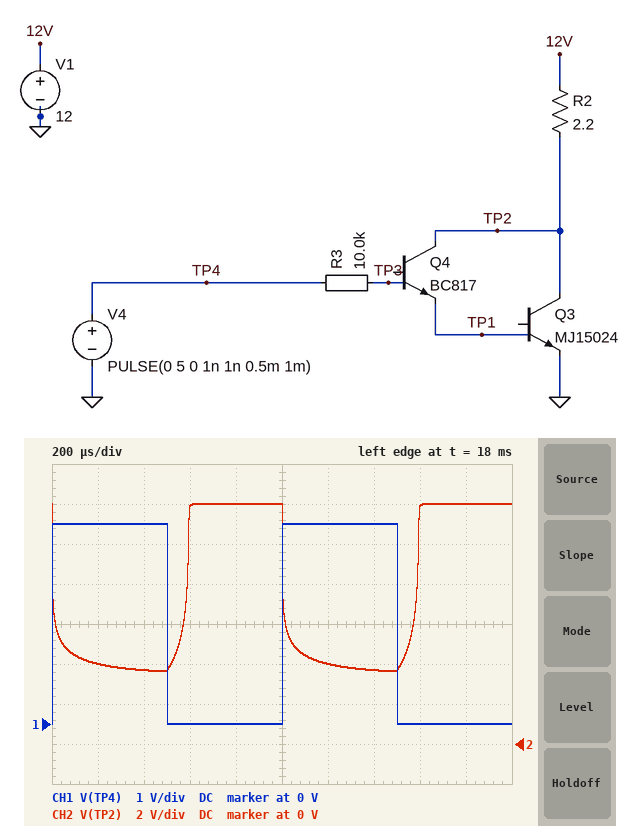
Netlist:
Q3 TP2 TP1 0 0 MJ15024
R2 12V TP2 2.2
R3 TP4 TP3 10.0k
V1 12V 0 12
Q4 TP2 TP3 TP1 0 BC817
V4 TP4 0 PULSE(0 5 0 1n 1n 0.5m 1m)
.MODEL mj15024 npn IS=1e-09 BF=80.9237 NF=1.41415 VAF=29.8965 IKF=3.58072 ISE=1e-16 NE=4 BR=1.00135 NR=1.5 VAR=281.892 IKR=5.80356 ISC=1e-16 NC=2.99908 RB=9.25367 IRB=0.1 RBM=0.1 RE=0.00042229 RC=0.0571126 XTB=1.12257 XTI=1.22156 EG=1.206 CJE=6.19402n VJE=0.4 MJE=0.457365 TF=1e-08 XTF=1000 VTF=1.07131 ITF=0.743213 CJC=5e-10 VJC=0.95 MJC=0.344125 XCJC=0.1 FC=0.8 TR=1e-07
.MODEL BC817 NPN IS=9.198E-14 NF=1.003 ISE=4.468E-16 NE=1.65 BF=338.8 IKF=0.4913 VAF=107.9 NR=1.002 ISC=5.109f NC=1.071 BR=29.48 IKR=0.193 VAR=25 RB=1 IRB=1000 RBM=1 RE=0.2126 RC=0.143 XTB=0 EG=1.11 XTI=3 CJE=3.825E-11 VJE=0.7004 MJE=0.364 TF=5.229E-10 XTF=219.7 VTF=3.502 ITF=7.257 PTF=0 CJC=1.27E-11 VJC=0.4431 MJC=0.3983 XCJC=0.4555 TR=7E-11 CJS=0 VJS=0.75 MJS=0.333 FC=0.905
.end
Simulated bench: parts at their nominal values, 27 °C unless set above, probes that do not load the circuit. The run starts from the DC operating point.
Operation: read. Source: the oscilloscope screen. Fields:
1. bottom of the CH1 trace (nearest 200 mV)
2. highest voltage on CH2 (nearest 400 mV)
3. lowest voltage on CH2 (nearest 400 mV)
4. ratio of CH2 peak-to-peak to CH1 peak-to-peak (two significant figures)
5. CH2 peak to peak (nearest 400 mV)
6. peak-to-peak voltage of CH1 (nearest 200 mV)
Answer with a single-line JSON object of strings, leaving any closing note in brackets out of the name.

{"bottom of the CH1 trace": "0 V", "highest voltage on CH2": "12.0 V", "lowest voltage on CH2": "3.6 V", "ratio of CH2 peak-to-peak to CH1 peak-to-peak": "1.7", "CH2 peak to peak": "8.4 V", "peak-to-peak voltage of CH1": "5.0 V"}
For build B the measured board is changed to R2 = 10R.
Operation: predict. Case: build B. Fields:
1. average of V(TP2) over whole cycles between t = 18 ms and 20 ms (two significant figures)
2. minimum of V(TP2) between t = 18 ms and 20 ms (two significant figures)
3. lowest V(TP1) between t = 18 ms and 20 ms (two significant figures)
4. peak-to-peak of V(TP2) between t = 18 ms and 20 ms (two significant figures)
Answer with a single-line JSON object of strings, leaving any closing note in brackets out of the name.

{"average of V(TP2) over whole cycles between t = 18 ms and 20 ms": "3.6 V", "minimum of V(TP2) between t = 18 ms and 20 ms": "940 mV", "lowest V(TP1) between t = 18 ms and 20 ms": "470 mV", "peak-to-peak of V(TP2) between t = 18 ms and 20 ms": "11 V"}
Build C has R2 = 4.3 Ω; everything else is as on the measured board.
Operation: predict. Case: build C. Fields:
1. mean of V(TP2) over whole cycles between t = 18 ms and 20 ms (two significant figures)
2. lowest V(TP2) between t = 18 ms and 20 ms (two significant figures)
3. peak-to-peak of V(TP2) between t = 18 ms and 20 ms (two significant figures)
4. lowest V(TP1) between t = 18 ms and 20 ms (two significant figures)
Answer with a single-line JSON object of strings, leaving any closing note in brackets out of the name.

{"mean of V(TP2) over whole cycles between t = 18 ms and 20 ms": "3.6 V", "lowest V(TP2) between t = 18 ms and 20 ms": "1.2 V", "peak-to-peak of V(TP2) between t = 18 ms and 20 ms": "11 V", "lowest V(TP1) between t = 18 ms and 20 ms": "490 mV"}
